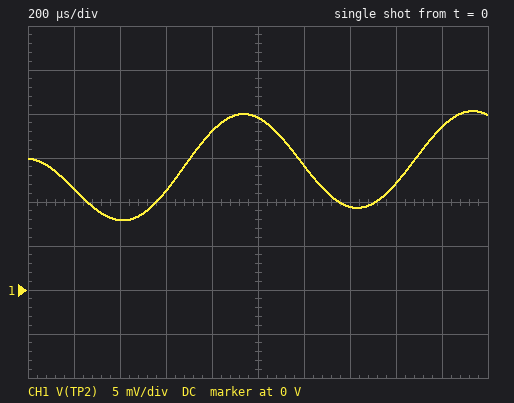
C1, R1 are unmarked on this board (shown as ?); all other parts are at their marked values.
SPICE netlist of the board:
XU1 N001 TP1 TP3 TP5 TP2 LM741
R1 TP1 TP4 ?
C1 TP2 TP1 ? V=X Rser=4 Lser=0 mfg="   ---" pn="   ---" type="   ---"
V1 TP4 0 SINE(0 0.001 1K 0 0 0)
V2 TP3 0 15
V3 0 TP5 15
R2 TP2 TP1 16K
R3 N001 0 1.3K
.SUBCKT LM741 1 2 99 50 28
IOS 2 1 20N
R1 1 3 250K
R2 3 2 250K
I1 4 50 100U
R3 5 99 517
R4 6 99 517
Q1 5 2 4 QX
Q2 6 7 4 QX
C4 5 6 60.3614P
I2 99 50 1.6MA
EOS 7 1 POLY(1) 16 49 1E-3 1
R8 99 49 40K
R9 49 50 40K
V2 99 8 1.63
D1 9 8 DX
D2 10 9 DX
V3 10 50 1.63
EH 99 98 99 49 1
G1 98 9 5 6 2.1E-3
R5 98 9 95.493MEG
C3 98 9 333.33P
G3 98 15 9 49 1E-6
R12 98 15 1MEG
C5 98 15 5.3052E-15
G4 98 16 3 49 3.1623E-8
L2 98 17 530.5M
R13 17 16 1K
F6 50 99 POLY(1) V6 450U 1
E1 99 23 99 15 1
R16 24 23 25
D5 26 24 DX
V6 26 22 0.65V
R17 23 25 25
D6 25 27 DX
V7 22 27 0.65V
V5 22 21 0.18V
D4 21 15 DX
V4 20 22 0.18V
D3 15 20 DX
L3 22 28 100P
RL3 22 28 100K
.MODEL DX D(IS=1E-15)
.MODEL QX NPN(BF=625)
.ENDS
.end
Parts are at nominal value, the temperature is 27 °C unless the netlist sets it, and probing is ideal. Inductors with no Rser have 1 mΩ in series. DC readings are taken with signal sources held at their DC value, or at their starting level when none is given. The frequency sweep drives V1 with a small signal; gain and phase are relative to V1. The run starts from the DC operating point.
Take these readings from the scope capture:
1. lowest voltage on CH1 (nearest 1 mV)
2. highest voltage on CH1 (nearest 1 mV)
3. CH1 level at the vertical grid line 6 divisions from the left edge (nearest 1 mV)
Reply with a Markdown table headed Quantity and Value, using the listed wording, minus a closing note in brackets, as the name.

| Quantity | Value |
|---|---|
| lowest voltage on CH1 | 8 mV |
| highest voltage on CH1 | 20 mV |
| CH1 level at the vertical grid line 6 divisions from the left edge | 14 mV |
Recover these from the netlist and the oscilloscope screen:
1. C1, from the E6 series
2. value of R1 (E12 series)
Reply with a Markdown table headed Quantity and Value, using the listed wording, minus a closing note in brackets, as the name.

| Quantity | Value |
|---|---|
| C1, from the E6 series | 22 nF |
| value of R1 | 1.2 kΩ |
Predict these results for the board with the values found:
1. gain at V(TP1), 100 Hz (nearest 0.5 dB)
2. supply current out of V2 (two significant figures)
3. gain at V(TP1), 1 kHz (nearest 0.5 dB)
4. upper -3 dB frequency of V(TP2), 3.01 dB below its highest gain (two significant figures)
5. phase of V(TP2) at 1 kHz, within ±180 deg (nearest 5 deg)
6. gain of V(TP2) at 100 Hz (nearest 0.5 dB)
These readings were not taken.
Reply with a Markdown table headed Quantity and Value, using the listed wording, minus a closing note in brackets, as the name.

| Quantity | Value |
|---|---|
| gain at V(TP1), 100 Hz | -57.5 dB |
| supply current out of V2 | 1.7 mA |
| gain at V(TP1), 1 kHz | -45.0 dB |
| upper -3 dB frequency of V(TP2), 3.01 dB below its highest gain | 450 Hz |
| phase of V(TP2) at 1 kHz, within ±180 deg | 115 deg |
| gain of V(TP2) at 100 Hz | 22.5 dB |
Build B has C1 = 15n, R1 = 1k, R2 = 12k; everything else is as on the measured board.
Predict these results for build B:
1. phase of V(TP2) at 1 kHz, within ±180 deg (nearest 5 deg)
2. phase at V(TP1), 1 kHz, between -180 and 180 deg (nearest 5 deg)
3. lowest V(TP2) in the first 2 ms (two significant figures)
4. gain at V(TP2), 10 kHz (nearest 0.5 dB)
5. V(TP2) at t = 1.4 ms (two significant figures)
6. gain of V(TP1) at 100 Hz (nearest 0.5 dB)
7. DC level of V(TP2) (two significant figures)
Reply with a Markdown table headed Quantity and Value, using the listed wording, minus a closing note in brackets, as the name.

| Quantity | Value |
|---|---|
| phase of V(TP2) at 1 kHz, within ±180 deg | 130 deg |
| phase at V(TP1), 1 kHz, between -180 and 180 deg | 40 deg |
| lowest V(TP2) in the first 2 ms | 4.6 mV |
| gain at V(TP2), 10 kHz | 0.5 dB |
| V(TP2) at t = 1.4 ms | 5.4 mV |
| gain of V(TP1) at 100 Hz | -58.5 dB |
| DC level of V(TP2) | 13 mV |
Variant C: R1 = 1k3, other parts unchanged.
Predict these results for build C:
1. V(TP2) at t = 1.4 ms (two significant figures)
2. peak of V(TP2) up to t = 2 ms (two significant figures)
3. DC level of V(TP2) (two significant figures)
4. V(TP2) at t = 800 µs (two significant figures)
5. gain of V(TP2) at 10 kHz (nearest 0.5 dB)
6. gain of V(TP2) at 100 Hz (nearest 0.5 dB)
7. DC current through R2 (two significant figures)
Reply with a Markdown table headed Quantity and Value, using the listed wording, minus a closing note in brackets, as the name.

| Quantity | Value |
|---|---|
| V(TP2) at t = 1.4 ms | 8.9 mV |
| peak of V(TP2) up to t = 2 ms | 19 mV |
| DC level of V(TP2) | 14 mV |
| V(TP2) at t = 800 µs | 17 mV |
| gain of V(TP2) at 10 kHz | -5.0 dB |
| gain of V(TP2) at 100 Hz | 21.5 dB |
| DC current through R2 | 810 nA |
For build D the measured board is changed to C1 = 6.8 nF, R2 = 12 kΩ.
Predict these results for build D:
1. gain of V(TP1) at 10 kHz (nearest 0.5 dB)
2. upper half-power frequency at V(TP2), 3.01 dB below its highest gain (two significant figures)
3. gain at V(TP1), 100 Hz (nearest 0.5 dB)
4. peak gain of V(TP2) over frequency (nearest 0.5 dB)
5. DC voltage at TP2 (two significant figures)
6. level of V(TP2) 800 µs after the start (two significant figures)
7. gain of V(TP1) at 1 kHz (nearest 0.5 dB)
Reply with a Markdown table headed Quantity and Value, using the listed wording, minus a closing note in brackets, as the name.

| Quantity | Value |
|---|---|
| gain of V(TP1) at 10 kHz | -34.5 dB |
| upper half-power frequency at V(TP2), 3.01 dB below its highest gain | 1.9 kHz |
| gain at V(TP1), 100 Hz | -60.0 dB |
| peak gain of V(TP2) over frequency | 20.0 dB |
| DC voltage at TP2 | 11 mV |
| level of V(TP2) 800 µs after the start | 20 mV |
| gain of V(TP1) at 1 kHz | -41.0 dB |
